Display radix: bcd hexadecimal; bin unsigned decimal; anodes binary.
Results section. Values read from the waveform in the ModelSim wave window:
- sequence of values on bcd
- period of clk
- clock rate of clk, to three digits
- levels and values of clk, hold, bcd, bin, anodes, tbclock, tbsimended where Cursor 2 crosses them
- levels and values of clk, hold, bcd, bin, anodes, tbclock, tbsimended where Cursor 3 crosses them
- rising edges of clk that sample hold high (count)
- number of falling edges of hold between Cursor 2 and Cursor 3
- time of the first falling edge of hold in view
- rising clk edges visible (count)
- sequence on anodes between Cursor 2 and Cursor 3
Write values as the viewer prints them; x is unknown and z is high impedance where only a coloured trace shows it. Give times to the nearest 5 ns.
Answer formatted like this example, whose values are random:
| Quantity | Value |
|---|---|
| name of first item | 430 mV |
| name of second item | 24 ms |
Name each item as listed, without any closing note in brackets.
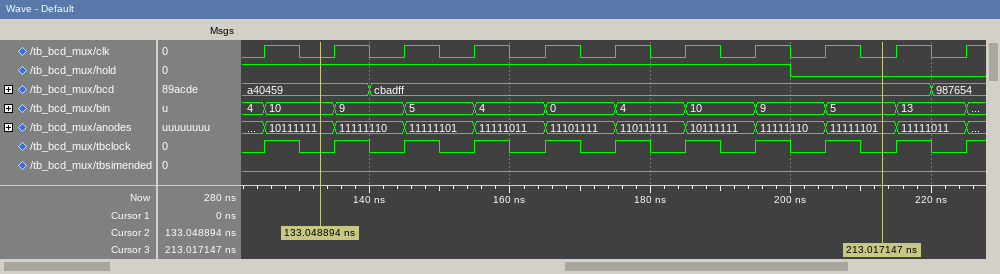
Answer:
| Quantity | Value |
|---|---|
| sequence of values on bcd | a40459, cbadff, 987654 |
| period of clk | 10 ns |
| clock rate of clk, to three digits | 100 MHz |
| levels and values of clk, hold, bcd, bin, anodes, tbclock, tbsimended where Cursor 2 crosses them | clk=0, hold=1, bcd=a40459, bin=10, anodes=10111111, tbclock=0, tbsimended=0 |
| levels and values of clk, hold, bcd, bin, anodes, tbclock, tbsimended where Cursor 3 crosses them | clk=0, hold=0, bcd=cbadff, bin=5, anodes=11111101, tbclock=0, tbsimended=0 |
| rising edges of clk that sample hold high | 8 |
| number of falling edges of hold between Cursor 2 and Cursor 3 | 1 |
| time of the first falling edge of hold in view | 200 ns |
| rising clk edges visible | 11 |
| sequence on anodes between Cursor 2 and Cursor 3 | 10111111, 11111110, 11111101, 11111011, 11101111, 11011111, 10111111, 11111110, 11111101 |
